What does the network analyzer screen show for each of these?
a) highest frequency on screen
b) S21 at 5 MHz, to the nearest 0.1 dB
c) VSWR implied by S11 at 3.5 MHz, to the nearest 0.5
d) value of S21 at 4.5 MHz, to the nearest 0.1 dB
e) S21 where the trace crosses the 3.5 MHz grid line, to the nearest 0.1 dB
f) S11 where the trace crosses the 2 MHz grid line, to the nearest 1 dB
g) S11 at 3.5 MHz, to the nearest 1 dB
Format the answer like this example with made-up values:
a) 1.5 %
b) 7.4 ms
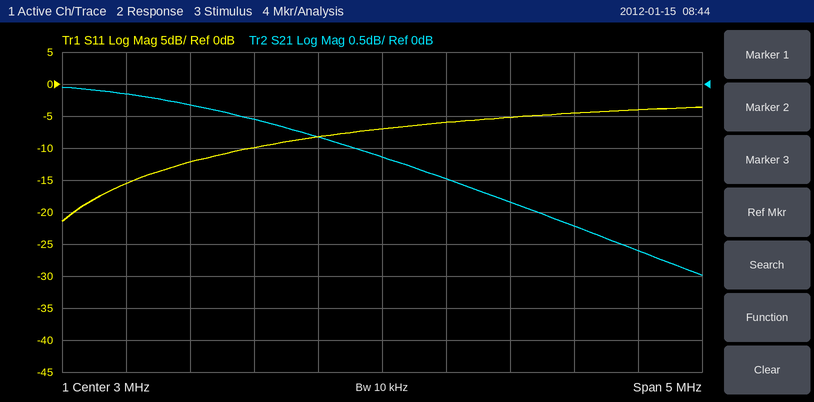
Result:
a) 5.5 MHz
b) -2.6 dB
c) 3.0
d) -2.2 dB
e) -1.5 dB
f) -10 dB
g) -6 dB
